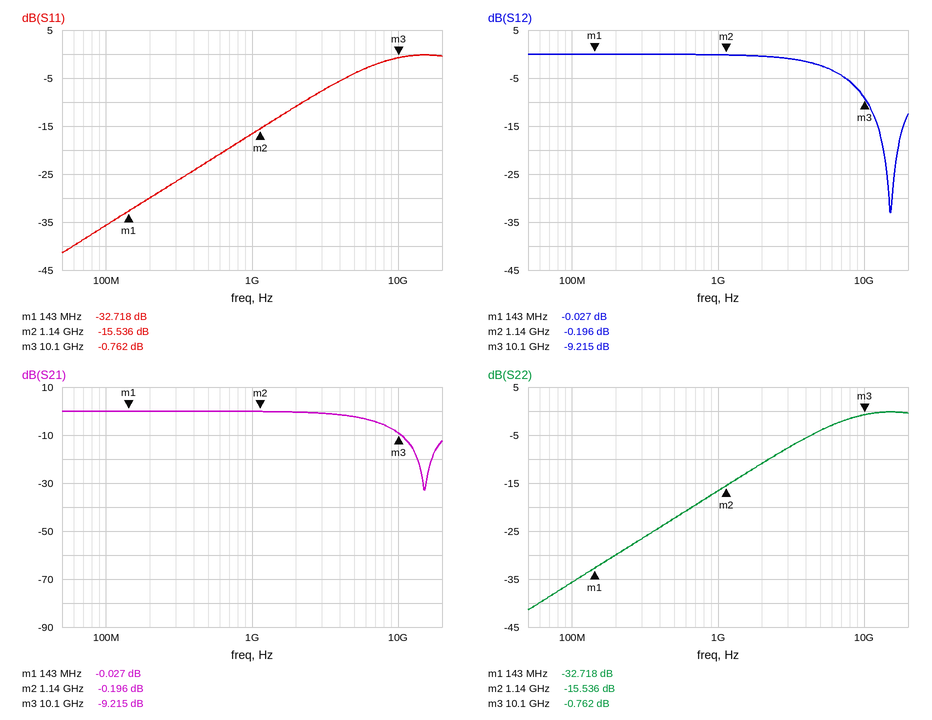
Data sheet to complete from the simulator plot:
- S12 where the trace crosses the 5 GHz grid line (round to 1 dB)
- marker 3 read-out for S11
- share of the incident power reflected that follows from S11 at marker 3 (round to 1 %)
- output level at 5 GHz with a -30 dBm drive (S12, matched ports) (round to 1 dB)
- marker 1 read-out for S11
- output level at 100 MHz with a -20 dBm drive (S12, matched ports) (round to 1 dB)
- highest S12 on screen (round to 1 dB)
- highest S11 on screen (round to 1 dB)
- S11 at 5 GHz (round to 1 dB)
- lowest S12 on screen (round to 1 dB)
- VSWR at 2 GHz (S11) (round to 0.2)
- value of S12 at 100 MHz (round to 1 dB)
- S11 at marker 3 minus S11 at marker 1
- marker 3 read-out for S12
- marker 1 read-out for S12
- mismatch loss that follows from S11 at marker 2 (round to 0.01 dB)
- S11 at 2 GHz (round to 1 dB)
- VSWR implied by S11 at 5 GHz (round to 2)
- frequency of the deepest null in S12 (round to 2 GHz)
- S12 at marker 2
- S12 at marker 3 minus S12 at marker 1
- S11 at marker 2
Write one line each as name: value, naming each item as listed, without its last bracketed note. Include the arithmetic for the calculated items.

S12 where the trace crosses the 5 GHz grid line: -2 dB
marker 3 read-out for S11: -0.762 dB
share of the incident power reflected that follows from S11 at marker 3: 10^(-0.762/10) ≈ 84 %
output level at 5 GHz with a -30 dBm drive (S12, matched ports): -30 dBm + (-2 dB) = -32 dBm
marker 1 read-out for S11: -32.718 dB
output level at 100 MHz with a -20 dBm drive (S12, matched ports): -20 dBm + (0 dB) = -20 dBm
highest S12 on screen: 0 dB
highest S11 on screen: 0 dB
S11 at 5 GHz: -4 dB
lowest S12 on screen: -33 dB
VSWR at 2 GHz (S11): |Γ| = 10^(-11/20) = 0.2818; VSWR = (1 + 0.2818)/(1 − 0.2818) ≈ 1.8
value of S12 at 100 MHz: 0 dB
S11 at marker 3 minus S11 at marker 1: -0.762 − (-32.718) = 31.956 dB
marker 3 read-out for S12: -9.215 dB
marker 1 read-out for S12: -0.027 dB
mismatch loss that follows from S11 at marker 2: −10 log10(1 − 10^(-15.536/10)) ≈ 0.12 dB
S11 at 2 GHz: -11 dB
VSWR implied by S11 at 5 GHz: |Γ| = 10^(-4/20) = 0.6310; VSWR = (1 + 0.6310)/(1 − 0.6310) ≈ 4
frequency of the deepest null in S12: 16 GHz
S12 at marker 2: -0.196 dB
S12 at marker 3 minus S12 at marker 1: -9.215 − (-0.027) = -9.188 dB
S11 at marker 2: -15.536 dB
